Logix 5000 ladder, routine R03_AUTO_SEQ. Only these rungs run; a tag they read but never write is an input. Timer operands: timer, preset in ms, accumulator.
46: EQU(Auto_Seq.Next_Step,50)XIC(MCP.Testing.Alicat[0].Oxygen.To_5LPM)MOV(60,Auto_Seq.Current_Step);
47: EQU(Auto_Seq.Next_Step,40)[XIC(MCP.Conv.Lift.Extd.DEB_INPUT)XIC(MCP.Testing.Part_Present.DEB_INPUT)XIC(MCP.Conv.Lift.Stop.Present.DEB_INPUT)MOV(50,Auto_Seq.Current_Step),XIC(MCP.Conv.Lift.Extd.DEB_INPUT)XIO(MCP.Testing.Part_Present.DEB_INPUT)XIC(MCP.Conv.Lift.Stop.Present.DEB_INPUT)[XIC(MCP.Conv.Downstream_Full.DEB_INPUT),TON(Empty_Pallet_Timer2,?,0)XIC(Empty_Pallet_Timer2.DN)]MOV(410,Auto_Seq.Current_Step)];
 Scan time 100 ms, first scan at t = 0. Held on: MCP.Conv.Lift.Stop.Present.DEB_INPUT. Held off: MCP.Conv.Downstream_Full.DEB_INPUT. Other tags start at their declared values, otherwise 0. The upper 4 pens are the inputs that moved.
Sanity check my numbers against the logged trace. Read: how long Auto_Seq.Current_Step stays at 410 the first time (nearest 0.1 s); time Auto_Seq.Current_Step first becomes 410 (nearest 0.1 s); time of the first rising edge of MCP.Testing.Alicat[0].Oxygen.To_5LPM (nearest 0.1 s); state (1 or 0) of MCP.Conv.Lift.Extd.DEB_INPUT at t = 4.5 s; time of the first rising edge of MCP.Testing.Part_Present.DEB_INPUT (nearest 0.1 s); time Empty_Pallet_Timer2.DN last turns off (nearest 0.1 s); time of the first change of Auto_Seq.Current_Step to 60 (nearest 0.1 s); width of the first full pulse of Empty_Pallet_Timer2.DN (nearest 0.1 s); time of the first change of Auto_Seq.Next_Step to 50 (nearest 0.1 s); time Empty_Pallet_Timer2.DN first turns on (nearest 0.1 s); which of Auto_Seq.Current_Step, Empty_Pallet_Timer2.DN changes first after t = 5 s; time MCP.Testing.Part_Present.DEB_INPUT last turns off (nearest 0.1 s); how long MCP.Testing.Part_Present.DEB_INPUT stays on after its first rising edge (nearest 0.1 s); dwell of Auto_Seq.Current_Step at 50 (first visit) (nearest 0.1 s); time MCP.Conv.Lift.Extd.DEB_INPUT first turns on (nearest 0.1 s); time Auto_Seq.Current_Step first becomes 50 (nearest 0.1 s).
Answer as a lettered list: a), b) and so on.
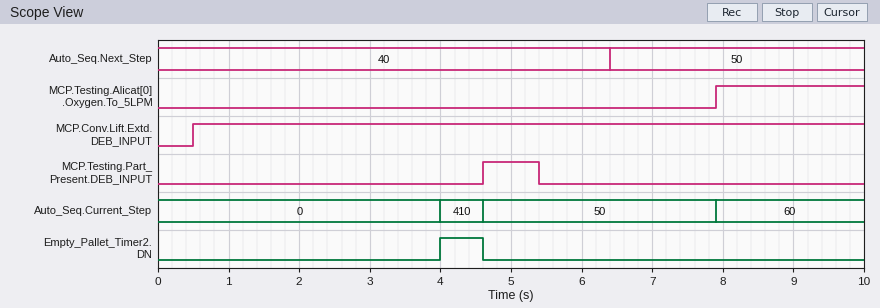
a) 0.6 s
b) 4.0 s
c) 7.9 s
d) 1
e) 4.6 s
f) 4.6 s
g) 7.9 s
h) 0.6 s
i) 6.4 s
j) 4.0 s
k) Auto_Seq.Current_Step
l) 5.4 s
m) 0.8 s
n) 3.3 s
o) 0.5 s
p) 4.6 s
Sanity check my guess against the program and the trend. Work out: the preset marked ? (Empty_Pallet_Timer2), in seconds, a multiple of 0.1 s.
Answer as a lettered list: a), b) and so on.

a) 3.5 s
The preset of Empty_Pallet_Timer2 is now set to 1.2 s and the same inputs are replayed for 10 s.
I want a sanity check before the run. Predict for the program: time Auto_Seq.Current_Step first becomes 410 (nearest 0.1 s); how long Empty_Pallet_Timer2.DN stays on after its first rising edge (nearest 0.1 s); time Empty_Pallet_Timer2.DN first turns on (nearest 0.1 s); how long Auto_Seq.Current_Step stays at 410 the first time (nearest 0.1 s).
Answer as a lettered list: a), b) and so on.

a) 1.7 s
b) 2.9 s
c) 1.7 s
d) 2.9 s
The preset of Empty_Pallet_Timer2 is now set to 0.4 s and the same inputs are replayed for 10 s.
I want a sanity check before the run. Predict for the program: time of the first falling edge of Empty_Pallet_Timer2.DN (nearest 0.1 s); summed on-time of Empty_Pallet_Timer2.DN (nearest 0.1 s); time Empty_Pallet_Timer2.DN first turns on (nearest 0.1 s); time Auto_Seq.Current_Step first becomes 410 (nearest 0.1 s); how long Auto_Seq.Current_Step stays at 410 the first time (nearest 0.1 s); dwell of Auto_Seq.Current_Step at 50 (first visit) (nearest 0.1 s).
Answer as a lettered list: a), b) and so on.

a) 4.6 s
b) 4.3 s
c) 0.9 s
d) 0.9 s
e) 3.7 s
f) 1.2 s
